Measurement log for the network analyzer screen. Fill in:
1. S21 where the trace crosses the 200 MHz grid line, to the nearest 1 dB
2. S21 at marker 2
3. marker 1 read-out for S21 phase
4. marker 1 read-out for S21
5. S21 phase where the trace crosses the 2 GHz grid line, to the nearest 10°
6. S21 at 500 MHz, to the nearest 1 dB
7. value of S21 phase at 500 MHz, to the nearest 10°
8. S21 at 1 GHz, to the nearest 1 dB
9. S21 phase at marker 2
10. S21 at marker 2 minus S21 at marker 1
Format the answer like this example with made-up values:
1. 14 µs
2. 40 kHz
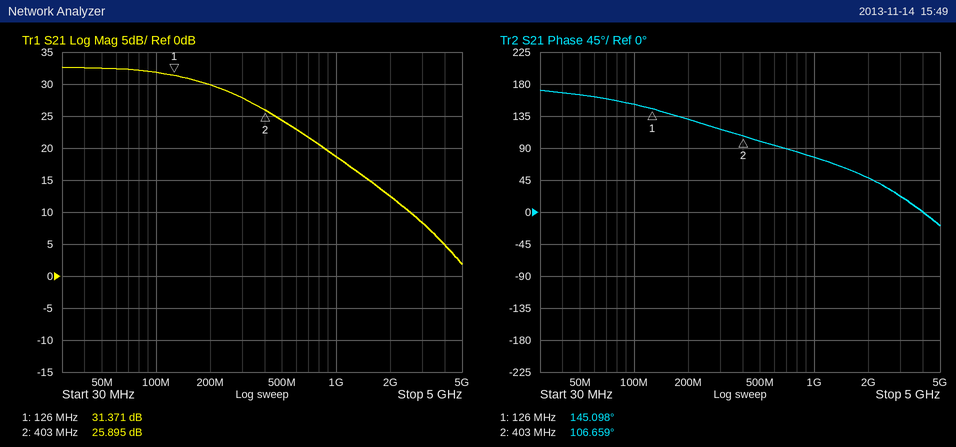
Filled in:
1. 30 dB
2. 25.895 dB
3. 145.098°
4. 31.371 dB
5. 50°
6. 24 dB
7. 100°
8. 19 dB
9. 106.659°
10. -5.476 dB
